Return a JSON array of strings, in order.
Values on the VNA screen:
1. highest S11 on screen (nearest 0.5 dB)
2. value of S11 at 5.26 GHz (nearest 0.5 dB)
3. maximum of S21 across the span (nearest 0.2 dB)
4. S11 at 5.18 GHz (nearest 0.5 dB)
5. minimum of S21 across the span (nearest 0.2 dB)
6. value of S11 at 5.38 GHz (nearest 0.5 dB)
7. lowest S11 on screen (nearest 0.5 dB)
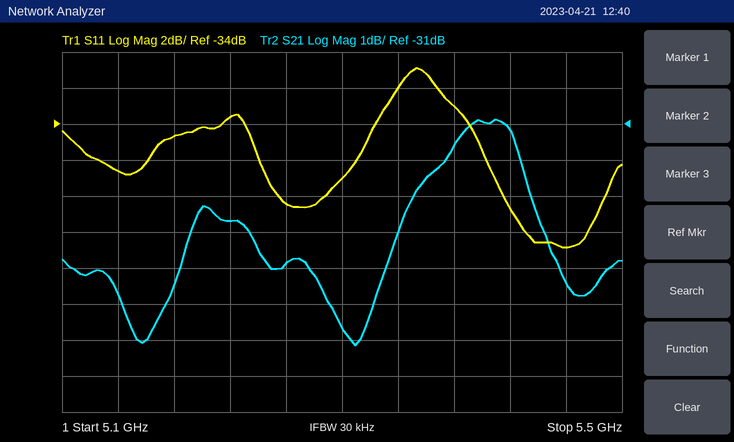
["-31.0 dB", "-38.5 dB", "-30.8 dB", "-34.5 dB", "-37.2 dB", "-33.0 dB", "-41.0 dB"]
